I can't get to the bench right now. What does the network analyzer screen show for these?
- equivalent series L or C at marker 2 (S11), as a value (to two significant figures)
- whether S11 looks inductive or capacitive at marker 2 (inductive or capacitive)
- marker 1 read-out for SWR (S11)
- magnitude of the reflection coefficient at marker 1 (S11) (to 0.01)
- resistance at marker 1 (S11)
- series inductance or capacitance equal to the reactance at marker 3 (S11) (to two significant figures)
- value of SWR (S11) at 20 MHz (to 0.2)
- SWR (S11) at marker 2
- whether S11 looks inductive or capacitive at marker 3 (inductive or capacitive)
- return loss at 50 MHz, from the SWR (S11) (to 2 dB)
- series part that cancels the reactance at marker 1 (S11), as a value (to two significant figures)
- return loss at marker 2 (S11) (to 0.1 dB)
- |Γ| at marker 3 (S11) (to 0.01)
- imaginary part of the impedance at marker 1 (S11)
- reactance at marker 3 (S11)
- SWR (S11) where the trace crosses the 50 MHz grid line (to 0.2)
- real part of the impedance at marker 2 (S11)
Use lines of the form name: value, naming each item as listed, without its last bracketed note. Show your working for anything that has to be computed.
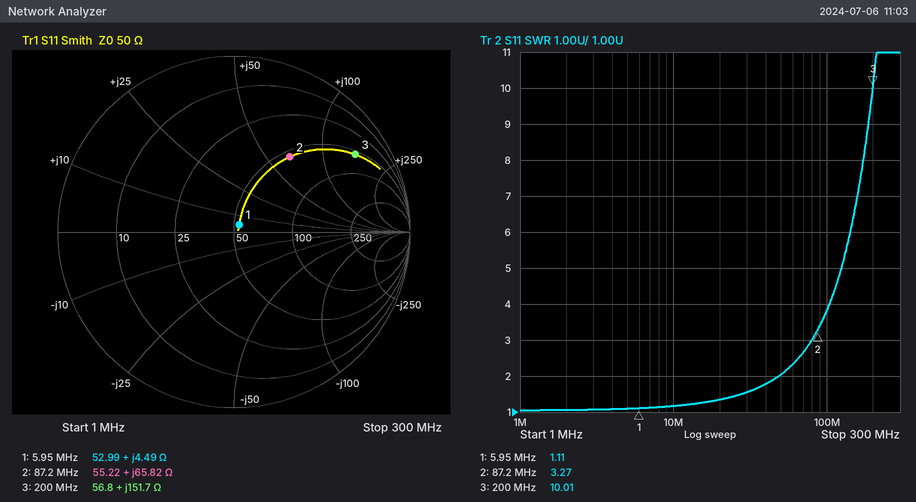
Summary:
equivalent series L or C at marker 2 (S11), as a value: L = 65.82 Ω/(2π × 87.2 MHz) ≈ 120 nH
whether S11 looks inductive or capacitive at marker 2: inductive
marker 1 read-out for SWR: 1.11
magnitude of the reflection coefficient at marker 1 (S11): 0.05
resistance at marker 1: 52.99 Ω
series inductance or capacitance equal to the reactance at marker 3 (S11): L = 151.7 Ω/(2π × 200 MHz) ≈ 121 nH, so 120 nH to two significant figures
value of SWR (S11) at 20 MHz: 1.4
SWR (S11) at marker 2: 3.27
whether S11 looks inductive or capacitive at marker 3: inductive
return loss at 50 MHz, from the SWR (S11): −20 log10((2 − 1)/(2 + 1)) ≈ 10 dB
series part that cancels the reactance at marker 1 (S11), as a value: C = 1/(2π × 5.95 MHz × 4.49 Ω) ≈ 6.0 nF
return loss at marker 2 (S11): 5.5 dB
|Γ| at marker 3 (S11): 0.82
imaginary part of the impedance at marker 1: +4.49 Ω
reactance at marker 3: +151.7 Ω
SWR (S11) where the trace crosses the 50 MHz grid line: 2.0
real part of the impedance at marker 2: 55.22 Ω
